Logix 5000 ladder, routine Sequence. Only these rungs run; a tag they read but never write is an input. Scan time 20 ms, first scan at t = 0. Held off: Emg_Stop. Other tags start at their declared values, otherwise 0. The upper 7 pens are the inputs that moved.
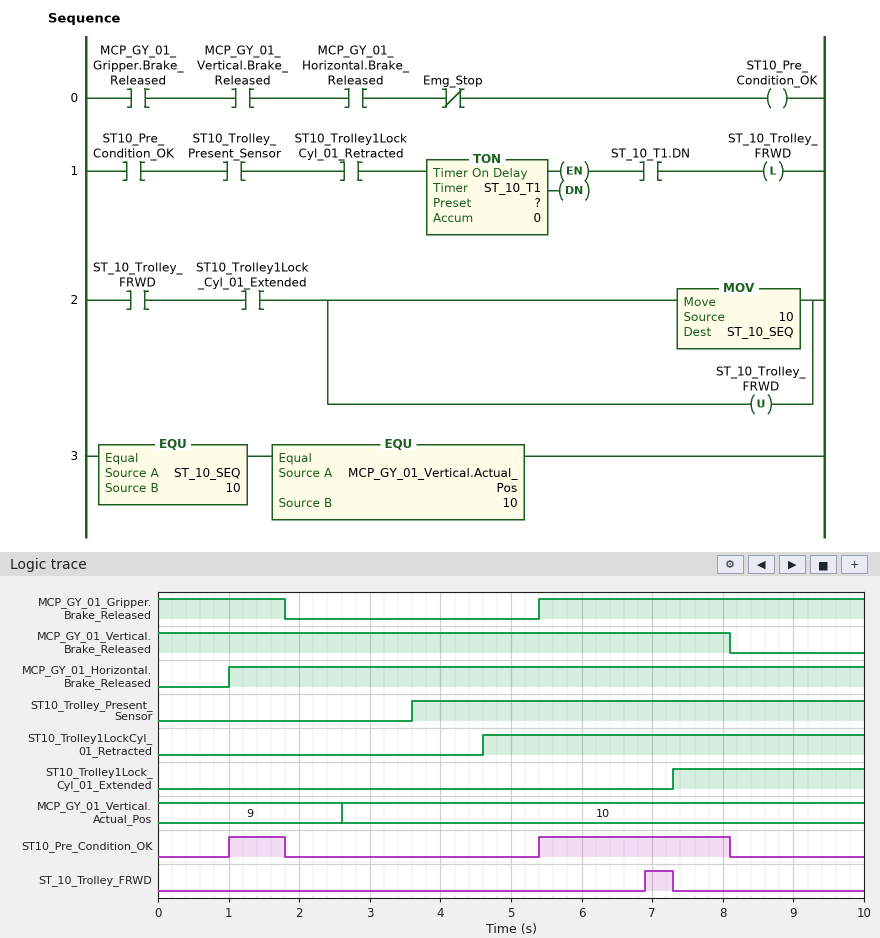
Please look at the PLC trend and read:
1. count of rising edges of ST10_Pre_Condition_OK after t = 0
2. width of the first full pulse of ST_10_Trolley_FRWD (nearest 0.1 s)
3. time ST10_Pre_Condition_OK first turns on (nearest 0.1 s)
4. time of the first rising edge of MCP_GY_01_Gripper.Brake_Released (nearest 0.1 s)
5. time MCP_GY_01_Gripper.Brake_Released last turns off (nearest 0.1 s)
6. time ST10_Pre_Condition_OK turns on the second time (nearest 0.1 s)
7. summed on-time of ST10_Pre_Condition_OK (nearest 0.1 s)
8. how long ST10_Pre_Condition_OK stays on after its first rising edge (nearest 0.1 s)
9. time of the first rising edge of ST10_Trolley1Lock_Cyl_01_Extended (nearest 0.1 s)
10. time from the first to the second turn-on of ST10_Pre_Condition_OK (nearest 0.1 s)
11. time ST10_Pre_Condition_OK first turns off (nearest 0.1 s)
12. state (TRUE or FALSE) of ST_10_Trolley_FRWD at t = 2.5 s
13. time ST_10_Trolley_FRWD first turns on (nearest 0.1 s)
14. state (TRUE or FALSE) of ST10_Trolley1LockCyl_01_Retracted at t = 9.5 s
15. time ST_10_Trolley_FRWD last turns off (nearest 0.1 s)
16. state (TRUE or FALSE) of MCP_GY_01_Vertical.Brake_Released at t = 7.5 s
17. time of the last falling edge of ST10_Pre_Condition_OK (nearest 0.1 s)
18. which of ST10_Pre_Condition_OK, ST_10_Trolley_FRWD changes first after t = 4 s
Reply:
2
0.4 s
1.0 s
5.4 s
1.8 s
5.4 s
3.5 s
0.8 s
7.3 s
4.4 s
1.8 s
FALSE
6.9 s
TRUE
7.3 s
TRUE
8.1 s
ST10_Pre_Condition_OK
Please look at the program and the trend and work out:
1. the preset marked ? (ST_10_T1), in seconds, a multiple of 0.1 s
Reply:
1.5 s
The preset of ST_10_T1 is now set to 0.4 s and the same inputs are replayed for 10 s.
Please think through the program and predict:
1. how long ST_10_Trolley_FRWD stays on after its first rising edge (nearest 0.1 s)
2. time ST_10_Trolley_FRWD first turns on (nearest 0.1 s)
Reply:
1.5 s
5.8 s
